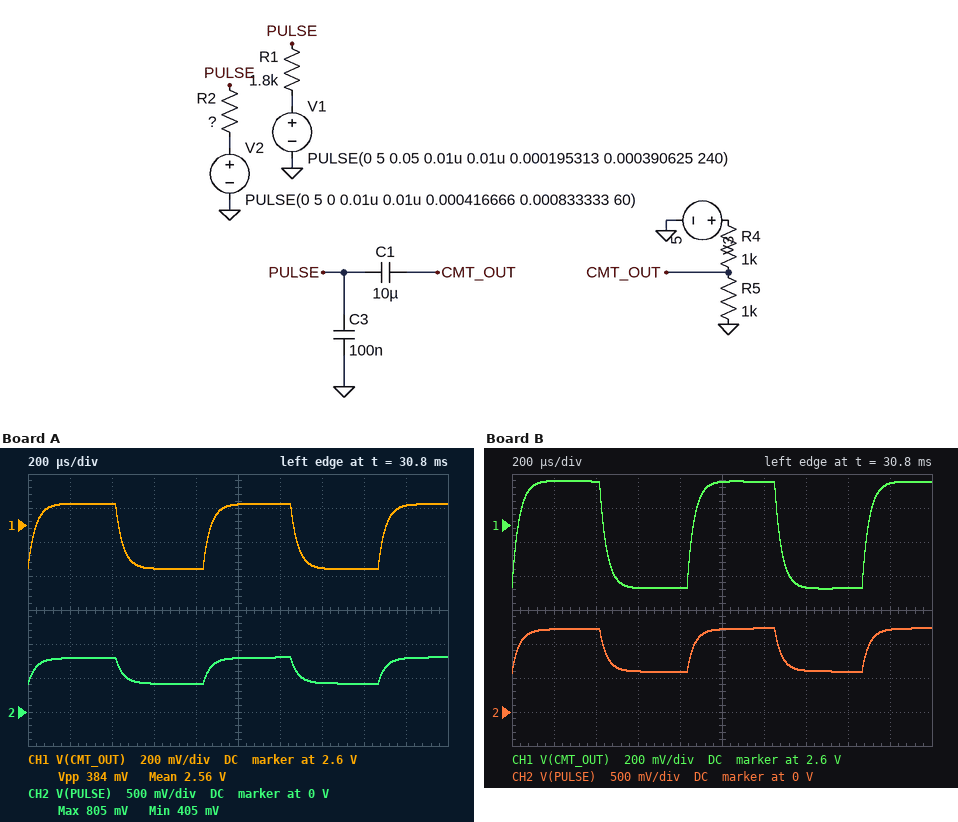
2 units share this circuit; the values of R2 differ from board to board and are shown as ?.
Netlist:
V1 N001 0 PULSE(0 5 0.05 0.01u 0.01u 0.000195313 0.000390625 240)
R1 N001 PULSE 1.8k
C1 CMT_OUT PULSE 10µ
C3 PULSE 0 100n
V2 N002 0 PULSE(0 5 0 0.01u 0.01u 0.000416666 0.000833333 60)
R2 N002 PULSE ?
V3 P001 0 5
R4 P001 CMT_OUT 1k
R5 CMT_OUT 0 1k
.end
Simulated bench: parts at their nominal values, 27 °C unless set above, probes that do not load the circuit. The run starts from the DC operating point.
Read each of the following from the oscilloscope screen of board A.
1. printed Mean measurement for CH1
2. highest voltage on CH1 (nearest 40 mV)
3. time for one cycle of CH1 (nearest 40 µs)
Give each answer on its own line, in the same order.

2.56 V
2.72 V
840 µs
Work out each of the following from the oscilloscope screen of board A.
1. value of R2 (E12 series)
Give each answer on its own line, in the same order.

4.7 kΩ
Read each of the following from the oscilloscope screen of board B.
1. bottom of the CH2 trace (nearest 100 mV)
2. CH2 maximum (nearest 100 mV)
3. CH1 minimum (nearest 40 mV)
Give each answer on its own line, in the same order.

600 mV
1.2 V
2.24 V
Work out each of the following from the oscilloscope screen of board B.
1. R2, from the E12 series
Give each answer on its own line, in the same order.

2.7 kΩ
